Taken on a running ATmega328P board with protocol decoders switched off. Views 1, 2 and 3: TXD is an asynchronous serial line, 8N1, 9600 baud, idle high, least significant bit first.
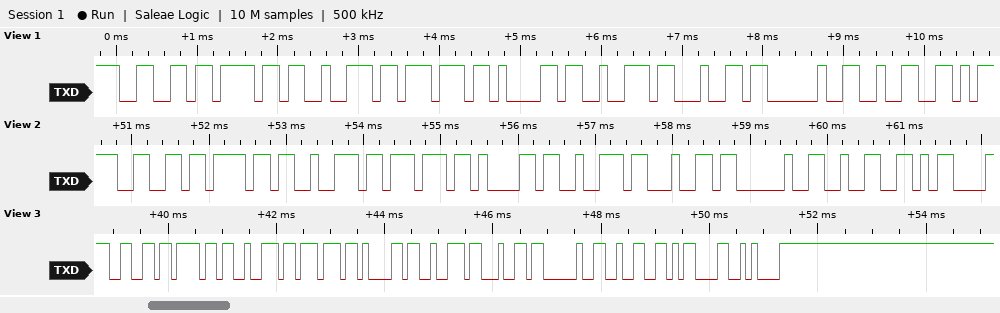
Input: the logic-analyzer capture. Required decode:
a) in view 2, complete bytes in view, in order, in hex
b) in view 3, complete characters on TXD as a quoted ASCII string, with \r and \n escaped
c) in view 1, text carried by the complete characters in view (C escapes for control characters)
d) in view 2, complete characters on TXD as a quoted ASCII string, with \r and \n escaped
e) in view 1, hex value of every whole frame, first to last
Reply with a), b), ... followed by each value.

a) 66 6F 72 77 61 72 64 20 32 0D
b) "forward 2\r\n"
c) "forward 2"
d) "forward 2\r"
e) 0x66 0x6F 0x72 0x77 0x61 0x72 0x64 0x20 0x32
